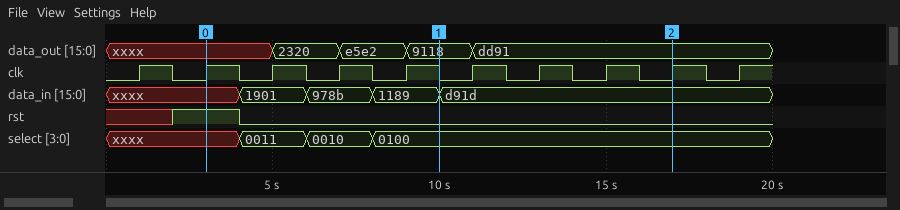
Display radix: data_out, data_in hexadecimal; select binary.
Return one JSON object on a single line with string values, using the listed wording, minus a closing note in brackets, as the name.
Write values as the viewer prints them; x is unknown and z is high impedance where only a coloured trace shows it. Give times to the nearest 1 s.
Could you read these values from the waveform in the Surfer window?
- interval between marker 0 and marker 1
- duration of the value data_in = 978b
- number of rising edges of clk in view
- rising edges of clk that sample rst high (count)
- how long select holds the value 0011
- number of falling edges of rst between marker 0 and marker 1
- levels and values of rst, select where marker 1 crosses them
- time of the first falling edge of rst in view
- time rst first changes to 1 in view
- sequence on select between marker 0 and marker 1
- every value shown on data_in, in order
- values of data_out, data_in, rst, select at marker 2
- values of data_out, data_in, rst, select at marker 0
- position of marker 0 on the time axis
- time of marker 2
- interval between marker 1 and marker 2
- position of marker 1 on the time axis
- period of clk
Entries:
{"interval between marker 0 and marker 1": "7 s", "duration of the value data_in = 978b": "2 s", "number of rising edges of clk in view": "10", "rising edges of clk that sample rst high": "1", "how long select holds the value 0011": "2 s", "number of falling edges of rst between marker 0 and marker 1": "1", "levels and values of rst, select where marker 1 crosses them": "rst=0, select=0100", "time of the first falling edge of rst in view": "4 s", "time rst first changes to 1 in view": "2 s", "sequence on select between marker 0 and marker 1": "xxxx, 0011, 0010, 0100", "every value shown on data_in, in order": "xxxx, 1901, 978b, 1189, d91d", "values of data_out, data_in, rst, select at marker 2": "data_out=dd91, data_in=d91d, rst=0, select=0100", "values of data_out, data_in, rst, select at marker 0": "data_out=xxxx, data_in=xxxx, rst=1, select=xxxx", "position of marker 0 on the time axis": "3 s", "time of marker 2": "17 s", "interval between marker 1 and marker 2": "7 s", "position of marker 1 on the time axis": "10 s", "period of clk": "2 s"}
